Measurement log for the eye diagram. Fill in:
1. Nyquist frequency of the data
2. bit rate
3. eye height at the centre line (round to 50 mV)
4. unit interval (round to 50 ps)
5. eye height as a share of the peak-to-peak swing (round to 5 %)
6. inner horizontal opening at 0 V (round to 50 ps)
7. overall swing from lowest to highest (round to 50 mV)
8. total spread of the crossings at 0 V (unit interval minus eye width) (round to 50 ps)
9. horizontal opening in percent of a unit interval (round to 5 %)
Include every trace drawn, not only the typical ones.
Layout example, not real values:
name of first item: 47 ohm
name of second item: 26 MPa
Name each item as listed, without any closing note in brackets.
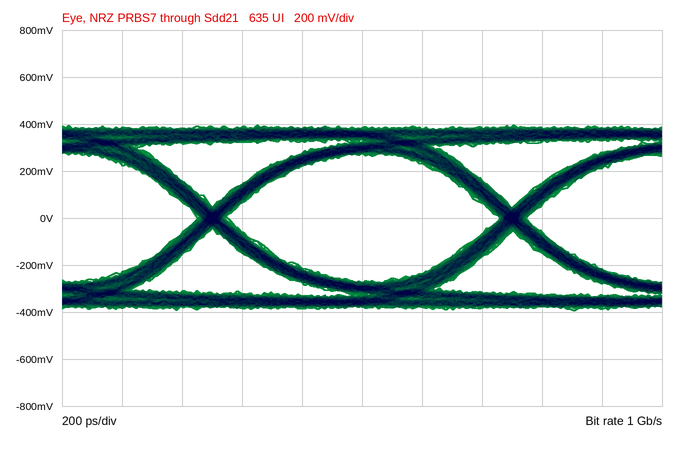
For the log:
Nyquist frequency of the data: 500 MHz
bit rate: 1 Gb/s
eye height at the centre line: 550 mV
unit interval: 1.00 ns
eye height as a share of the peak-to-peak swing: 70 %
inner horizontal opening at 0 V: 900 ps
overall swing from lowest to highest: 800 mV
total spread of the crossings at 0 V (unit interval minus eye width): 100 ps
horizontal opening in percent of a unit interval: 90 %
